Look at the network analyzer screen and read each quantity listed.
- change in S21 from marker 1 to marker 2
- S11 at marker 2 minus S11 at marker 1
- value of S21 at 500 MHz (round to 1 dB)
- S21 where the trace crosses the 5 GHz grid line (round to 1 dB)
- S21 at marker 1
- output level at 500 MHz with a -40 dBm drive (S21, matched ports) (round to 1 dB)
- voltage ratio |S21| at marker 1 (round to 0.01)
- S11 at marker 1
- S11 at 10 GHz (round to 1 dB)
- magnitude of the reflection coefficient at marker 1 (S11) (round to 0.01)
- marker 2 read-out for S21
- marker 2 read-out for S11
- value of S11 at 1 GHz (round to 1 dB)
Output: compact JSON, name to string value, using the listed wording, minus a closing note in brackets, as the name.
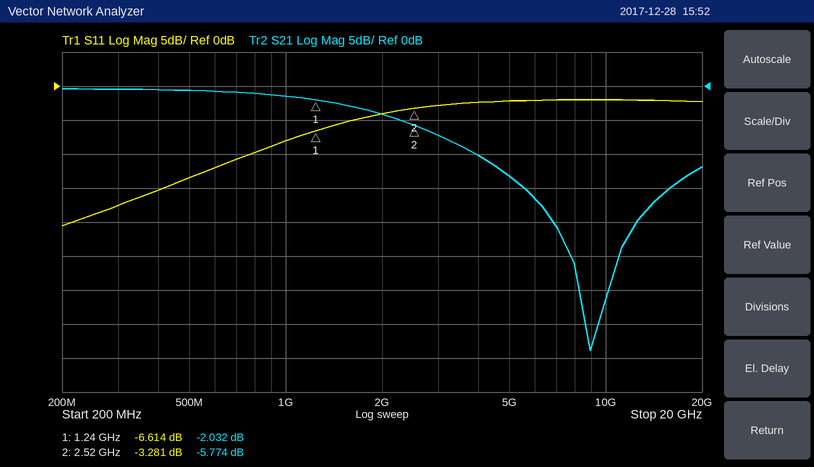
{"change in S21 from marker 1 to marker 2": "-3.742 dB", "S11 at marker 2 minus S11 at marker 1": "3.333 dB", "value of S21 at 500 MHz": "-1 dB", "S21 where the trace crosses the 5 GHz grid line": "-13 dB", "S21 at marker 1": "-2.032 dB", "output level at 500 MHz with a -40 dBm drive (S21, matched ports)": "-41 dBm", "voltage ratio |S21| at marker 1": "0.79", "S11 at marker 1": "-6.614 dB", "S11 at 10 GHz": "-2 dB", "magnitude of the reflection coefficient at marker 1 (S11)": "0.47", "marker 2 read-out for S21": "-5.774 dB", "marker 2 read-out for S11": "-3.281 dB", "value of S11 at 1 GHz": "-8 dB"}
